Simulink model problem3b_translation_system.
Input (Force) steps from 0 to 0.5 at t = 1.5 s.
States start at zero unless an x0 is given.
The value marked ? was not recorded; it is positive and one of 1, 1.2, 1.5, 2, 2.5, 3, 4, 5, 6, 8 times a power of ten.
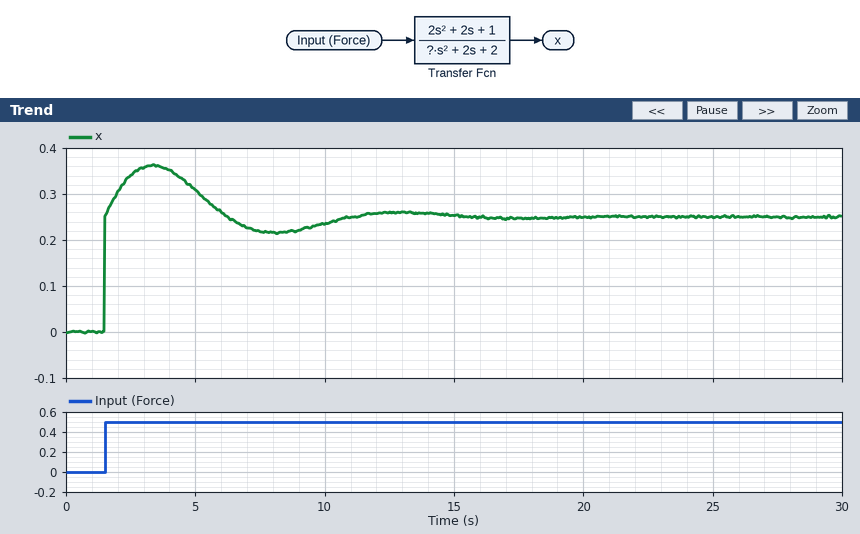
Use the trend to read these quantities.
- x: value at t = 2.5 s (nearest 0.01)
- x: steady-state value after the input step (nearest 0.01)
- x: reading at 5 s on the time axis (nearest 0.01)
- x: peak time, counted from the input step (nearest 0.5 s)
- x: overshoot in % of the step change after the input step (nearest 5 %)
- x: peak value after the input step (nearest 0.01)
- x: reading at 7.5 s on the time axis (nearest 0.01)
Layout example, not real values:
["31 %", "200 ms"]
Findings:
["0.34", "0.25", "0.31", "2.0 s", "45 %", "0.36", "0.22"]
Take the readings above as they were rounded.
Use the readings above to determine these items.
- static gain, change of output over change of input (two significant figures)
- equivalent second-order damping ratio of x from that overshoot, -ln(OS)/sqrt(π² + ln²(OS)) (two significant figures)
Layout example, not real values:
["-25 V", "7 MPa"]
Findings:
["0.50", "0.25"]
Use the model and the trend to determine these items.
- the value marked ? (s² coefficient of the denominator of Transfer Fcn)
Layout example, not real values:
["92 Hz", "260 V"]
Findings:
["4"]
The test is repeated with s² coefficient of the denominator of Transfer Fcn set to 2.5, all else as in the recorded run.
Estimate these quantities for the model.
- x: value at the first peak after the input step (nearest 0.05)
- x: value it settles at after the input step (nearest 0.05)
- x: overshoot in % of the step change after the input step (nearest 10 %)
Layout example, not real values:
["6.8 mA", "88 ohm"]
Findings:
["0.40", "0.25", "70 %"]
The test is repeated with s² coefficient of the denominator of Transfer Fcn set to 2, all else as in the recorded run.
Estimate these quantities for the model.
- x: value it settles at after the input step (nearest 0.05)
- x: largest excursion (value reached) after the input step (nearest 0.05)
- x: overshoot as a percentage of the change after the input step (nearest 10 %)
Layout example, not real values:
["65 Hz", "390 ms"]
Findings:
["0.25", "0.50", "100 %"]
